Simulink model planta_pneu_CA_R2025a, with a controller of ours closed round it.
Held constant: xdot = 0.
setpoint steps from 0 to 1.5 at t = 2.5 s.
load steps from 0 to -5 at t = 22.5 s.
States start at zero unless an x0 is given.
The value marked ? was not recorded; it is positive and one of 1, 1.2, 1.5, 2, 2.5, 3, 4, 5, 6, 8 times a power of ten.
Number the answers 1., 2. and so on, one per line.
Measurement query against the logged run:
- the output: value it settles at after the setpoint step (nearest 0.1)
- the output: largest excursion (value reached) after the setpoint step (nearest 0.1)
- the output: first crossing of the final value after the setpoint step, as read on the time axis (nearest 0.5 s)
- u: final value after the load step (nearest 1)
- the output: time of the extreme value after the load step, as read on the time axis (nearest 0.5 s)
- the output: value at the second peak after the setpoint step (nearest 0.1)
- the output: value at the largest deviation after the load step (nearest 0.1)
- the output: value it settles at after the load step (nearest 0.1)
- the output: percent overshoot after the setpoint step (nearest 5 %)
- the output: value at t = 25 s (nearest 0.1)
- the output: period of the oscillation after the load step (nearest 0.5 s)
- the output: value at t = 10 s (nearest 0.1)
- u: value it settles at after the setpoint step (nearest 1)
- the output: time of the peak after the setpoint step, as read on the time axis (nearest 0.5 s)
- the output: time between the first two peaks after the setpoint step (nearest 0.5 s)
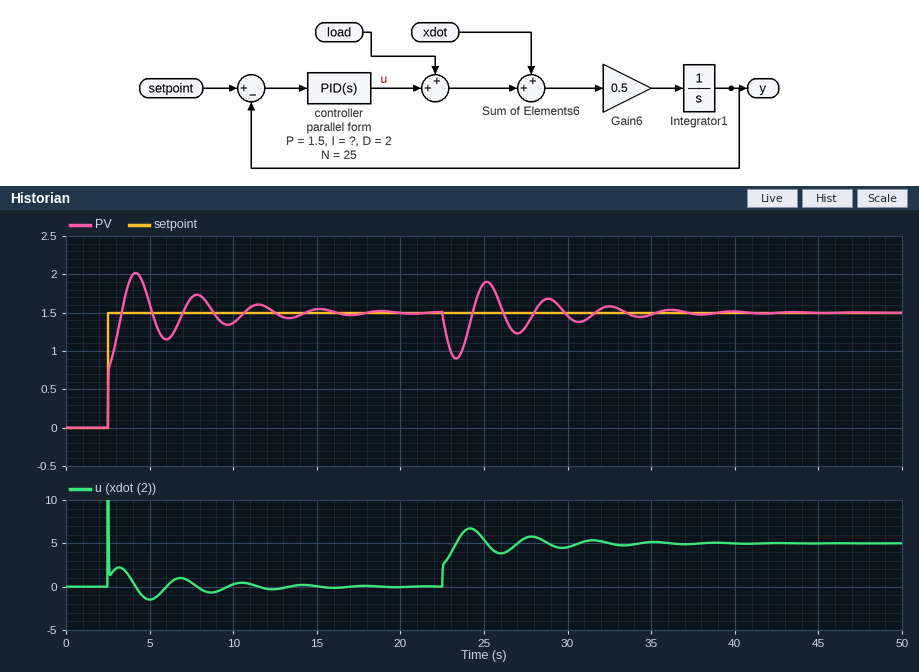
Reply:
1. 1.5
2. 2.0
3. 3.5 s
4. 5
5. 23.5 s
6. 1.7
7. 0.9
8. 1.5
9. 35 %
10. 1.9
11. 3.5 s
12. 1.4
13. 0
14. 4.0 s
15. 3.5 s
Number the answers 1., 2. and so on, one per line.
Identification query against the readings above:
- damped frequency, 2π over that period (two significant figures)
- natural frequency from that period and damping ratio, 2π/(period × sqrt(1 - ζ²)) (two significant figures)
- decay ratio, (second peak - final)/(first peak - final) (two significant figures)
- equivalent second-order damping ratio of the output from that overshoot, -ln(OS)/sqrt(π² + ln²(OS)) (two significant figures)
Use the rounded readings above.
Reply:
1. 1.8 rad/s
2. 1.9 rad/s
3. 0.40
4. 0.32
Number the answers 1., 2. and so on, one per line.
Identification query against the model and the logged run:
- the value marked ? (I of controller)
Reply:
1. 12
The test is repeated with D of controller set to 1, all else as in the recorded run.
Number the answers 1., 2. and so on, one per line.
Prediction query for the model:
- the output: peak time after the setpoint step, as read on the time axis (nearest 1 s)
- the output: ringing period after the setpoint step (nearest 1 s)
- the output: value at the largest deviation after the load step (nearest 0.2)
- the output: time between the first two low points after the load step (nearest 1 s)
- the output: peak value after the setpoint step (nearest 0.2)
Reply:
1. 4 s
2. 3 s
3. 0.8
4. 3 s
5. 2.2
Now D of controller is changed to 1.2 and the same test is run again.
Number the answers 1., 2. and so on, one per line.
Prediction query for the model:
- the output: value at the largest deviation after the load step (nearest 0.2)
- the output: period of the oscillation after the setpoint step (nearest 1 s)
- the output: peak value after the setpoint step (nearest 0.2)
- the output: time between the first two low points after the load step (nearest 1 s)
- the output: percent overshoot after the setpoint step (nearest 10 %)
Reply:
1. 0.8
2. 3 s
3. 2.2
4. 3 s
5. 40 %
